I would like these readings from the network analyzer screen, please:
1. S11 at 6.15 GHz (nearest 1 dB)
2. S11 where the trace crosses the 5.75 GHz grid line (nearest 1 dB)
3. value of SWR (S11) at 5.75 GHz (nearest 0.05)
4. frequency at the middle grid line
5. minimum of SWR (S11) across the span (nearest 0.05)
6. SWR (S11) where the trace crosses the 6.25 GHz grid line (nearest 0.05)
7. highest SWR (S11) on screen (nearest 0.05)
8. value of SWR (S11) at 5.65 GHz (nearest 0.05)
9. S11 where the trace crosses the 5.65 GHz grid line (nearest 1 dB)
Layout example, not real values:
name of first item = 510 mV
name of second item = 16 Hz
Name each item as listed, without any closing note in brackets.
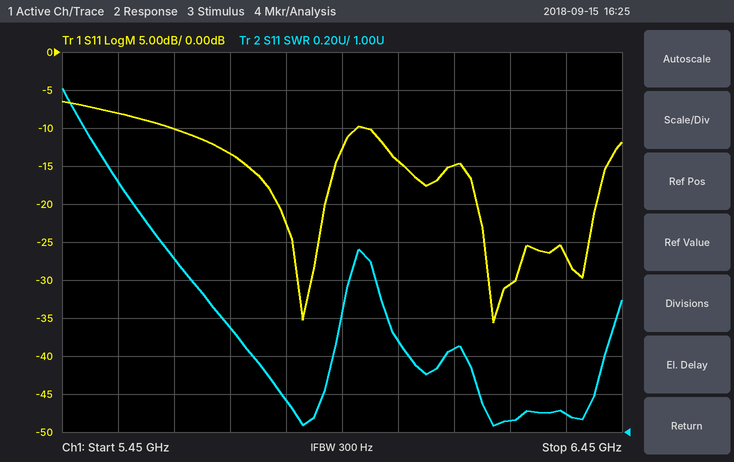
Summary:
S11 at 6.15 GHz = -15 dB
S11 where the trace crosses the 5.75 GHz grid line = -13 dB
value of SWR (S11) at 5.75 GHz = 1.55
frequency at the middle grid line = 5.95 GHz
minimum of SWR (S11) across the span = 1.05
SWR (S11) where the trace crosses the 6.25 GHz grid line = 1.05
highest SWR (S11) on screen = 2.80
value of SWR (S11) at 5.65 GHz = 1.90
S11 where the trace crosses the 5.65 GHz grid line = -10 dB
